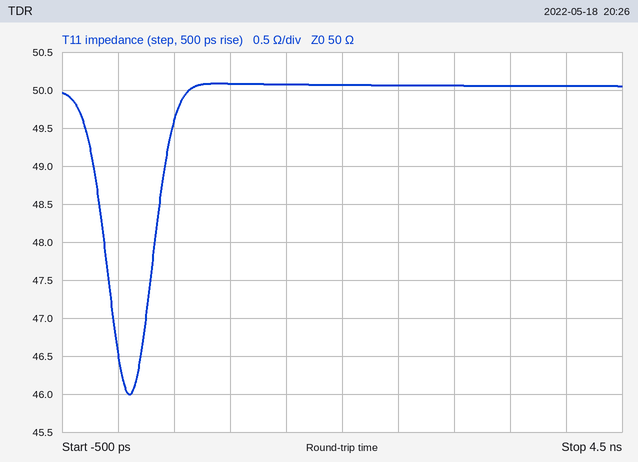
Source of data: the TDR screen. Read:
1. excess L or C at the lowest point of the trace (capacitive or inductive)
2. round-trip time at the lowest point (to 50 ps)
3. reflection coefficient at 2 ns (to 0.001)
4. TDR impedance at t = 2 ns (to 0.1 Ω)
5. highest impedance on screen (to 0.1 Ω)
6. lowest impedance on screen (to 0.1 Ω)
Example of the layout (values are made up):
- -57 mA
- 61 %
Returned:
- capacitive
- 100 ps
- +0.001
- 50.1 Ω
- 50.1 Ω
- 46.0 Ω
